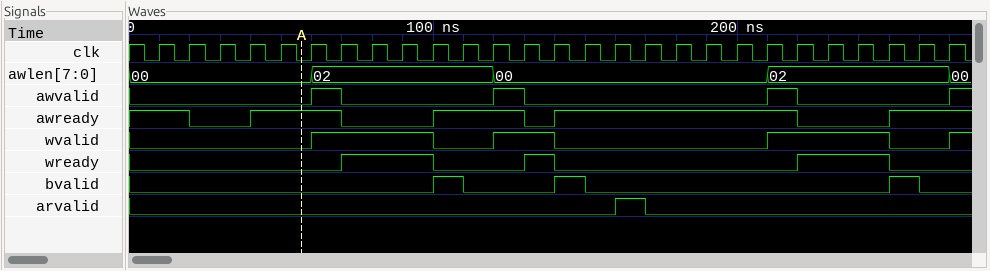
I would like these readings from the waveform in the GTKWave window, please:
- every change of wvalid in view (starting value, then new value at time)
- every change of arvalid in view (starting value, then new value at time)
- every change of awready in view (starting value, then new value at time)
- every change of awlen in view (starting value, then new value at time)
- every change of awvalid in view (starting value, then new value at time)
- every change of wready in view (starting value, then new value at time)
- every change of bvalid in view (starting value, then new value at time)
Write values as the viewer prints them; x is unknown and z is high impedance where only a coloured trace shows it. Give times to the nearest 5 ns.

0, 1 at 60 ns, 0 at 100 ns, 1 at 120 ns, 0 at 140 ns, 1 at 210 ns, 0 at 250 ns, 1 at 270 ns
0, 1 at 160 ns, 0 at 170 ns
1, 0 at 20 ns, 1 at 40 ns, 0 at 70 ns, 1 at 100 ns, 0 at 130 ns, 1 at 140 ns, 0 at 220 ns, 1 at 250 ns
00, 02 at 60 ns, 00 at 120 ns, 02 at 210 ns, 00 at 270 ns
0, 1 at 60 ns, 0 at 70 ns, 1 at 120 ns, 0 at 130 ns, 1 at 210 ns, 0 at 220 ns, 1 at 270 ns
0, 1 at 70 ns, 0 at 100 ns, 1 at 130 ns, 0 at 140 ns, 1 at 220 ns, 0 at 250 ns
0, 1 at 100 ns, 0 at 110 ns, 1 at 140 ns, 0 at 150 ns, 1 at 250 ns, 0 at 260 ns
